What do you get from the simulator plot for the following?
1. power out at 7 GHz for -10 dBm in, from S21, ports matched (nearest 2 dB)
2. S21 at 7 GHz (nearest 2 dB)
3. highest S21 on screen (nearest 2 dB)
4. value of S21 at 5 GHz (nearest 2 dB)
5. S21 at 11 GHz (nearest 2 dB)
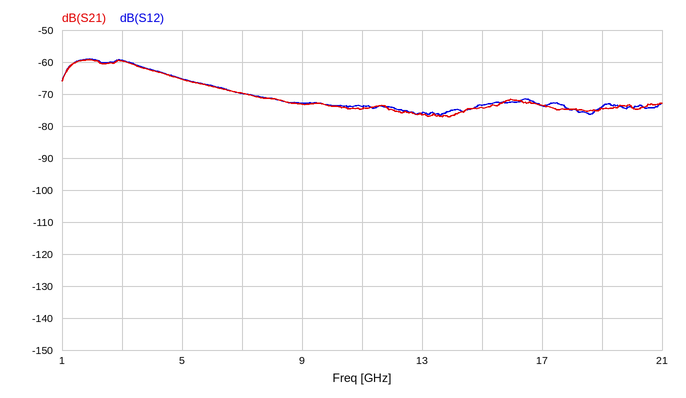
-80 dBm
-70 dB
-60 dB
-66 dB
-74 dB
